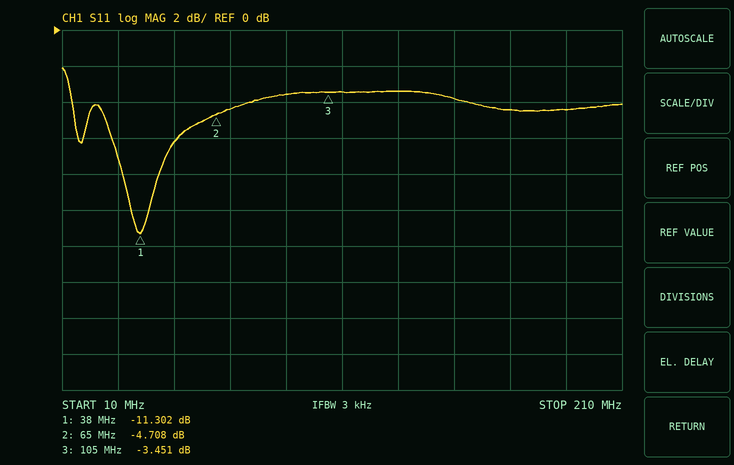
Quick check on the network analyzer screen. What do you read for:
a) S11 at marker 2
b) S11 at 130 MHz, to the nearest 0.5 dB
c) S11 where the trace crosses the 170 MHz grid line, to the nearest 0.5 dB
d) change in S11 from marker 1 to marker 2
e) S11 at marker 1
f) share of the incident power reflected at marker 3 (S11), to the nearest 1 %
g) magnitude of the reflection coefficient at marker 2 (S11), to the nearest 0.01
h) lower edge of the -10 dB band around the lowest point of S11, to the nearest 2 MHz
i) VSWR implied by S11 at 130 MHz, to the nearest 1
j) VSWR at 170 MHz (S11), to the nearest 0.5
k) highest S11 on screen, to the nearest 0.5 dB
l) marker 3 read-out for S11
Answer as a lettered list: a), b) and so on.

a) -4.708 dB
b) -3.5 dB
c) -4.5 dB
d) 6.594 dB
e) -11.302 dB
f) 45 %
g) 0.58
h) 34 MHz
i) 5
j) 4.0
k) -2.0 dB
l) -3.451 dB
